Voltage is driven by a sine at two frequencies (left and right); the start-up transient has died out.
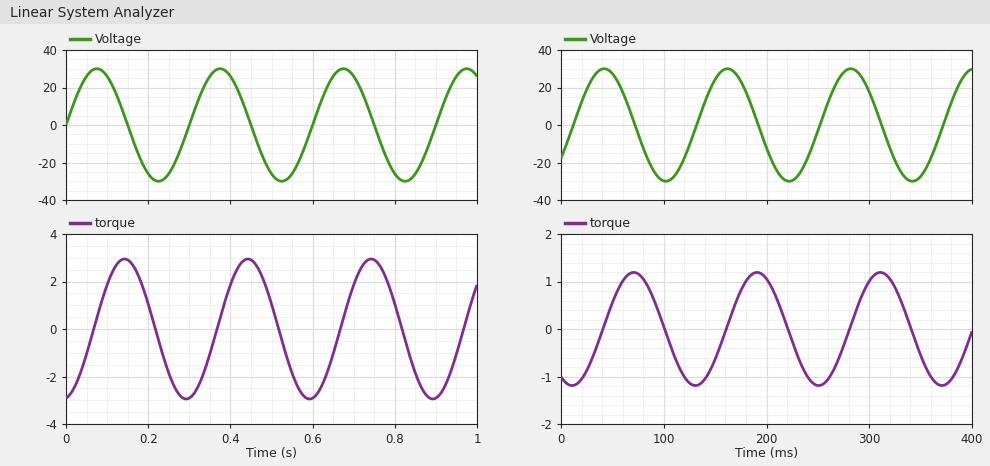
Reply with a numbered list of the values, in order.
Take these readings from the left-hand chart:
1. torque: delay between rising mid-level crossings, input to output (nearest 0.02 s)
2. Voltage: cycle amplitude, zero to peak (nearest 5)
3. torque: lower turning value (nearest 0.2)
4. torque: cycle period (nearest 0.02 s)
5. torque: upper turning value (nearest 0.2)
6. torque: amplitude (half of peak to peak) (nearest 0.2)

1. 0.06 s
2. 30
3. -3.0
4. 0.30 s
5. 3.0
6. 3.0
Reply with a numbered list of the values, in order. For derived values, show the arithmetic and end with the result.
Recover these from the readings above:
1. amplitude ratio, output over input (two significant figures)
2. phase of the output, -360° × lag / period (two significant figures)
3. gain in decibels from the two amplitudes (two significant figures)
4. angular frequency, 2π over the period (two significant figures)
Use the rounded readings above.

1. 3 / 30 = 0.10
2. -360 × 0.06 / 0.3 = -72°
3. 20 log10(3 / 30) = -20 dB
4. 2π / 0.3 = 21 rad/s
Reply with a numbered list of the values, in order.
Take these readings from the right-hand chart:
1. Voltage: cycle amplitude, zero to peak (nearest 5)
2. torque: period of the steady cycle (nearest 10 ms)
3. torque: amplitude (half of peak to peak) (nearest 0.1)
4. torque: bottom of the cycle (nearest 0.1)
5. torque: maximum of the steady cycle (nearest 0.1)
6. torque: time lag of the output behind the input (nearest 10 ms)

1. 30
2. 120 ms
3. 1.2
4. -1.2
5. 1.2
6. 30 ms
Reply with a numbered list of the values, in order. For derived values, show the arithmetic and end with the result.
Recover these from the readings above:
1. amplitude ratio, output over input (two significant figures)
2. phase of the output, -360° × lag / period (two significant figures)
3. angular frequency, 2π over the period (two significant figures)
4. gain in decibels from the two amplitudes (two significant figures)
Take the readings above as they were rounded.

1. 1.2 / 30 = 0.040
2. -360 × 30 / 120 = -90°
3. 2π / 120 = 0.052 rad/ms
4. 20 log10(1.2 / 30) = -28 dB
